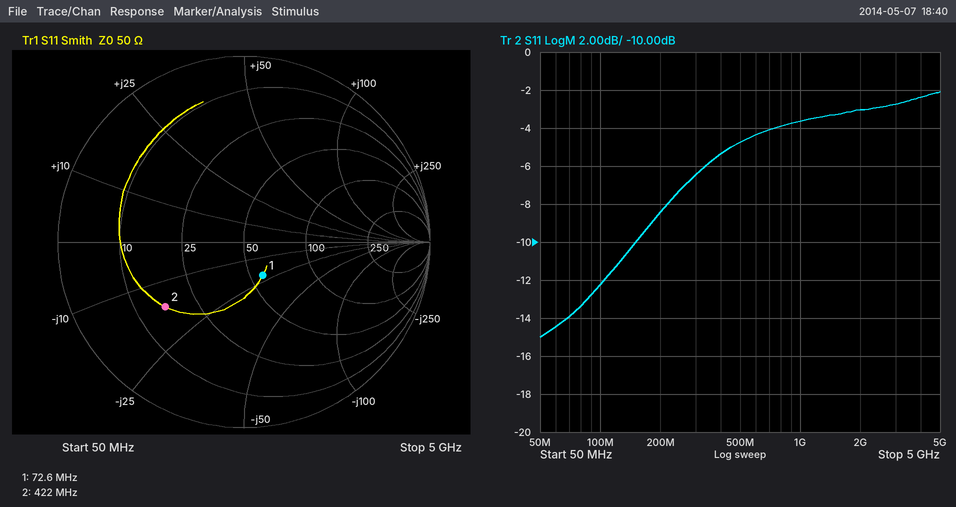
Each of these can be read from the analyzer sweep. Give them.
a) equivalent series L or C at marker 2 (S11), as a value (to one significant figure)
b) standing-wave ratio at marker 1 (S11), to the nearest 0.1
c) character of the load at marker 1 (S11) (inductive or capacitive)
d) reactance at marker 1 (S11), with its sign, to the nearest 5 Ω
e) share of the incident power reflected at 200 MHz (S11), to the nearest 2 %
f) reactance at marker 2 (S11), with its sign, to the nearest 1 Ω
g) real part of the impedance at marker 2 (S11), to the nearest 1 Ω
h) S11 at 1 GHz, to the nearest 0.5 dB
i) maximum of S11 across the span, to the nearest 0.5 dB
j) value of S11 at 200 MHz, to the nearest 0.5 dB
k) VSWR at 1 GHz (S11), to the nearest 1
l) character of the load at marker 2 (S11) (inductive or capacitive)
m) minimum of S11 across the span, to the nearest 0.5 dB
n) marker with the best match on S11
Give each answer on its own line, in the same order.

20 pF
1.5
capacitive
-20 Ω
14 %
-16 Ω
16 Ω
-3.5 dB
-2.0 dB
-8.5 dB
5
capacitive
-15.0 dB
marker 1
